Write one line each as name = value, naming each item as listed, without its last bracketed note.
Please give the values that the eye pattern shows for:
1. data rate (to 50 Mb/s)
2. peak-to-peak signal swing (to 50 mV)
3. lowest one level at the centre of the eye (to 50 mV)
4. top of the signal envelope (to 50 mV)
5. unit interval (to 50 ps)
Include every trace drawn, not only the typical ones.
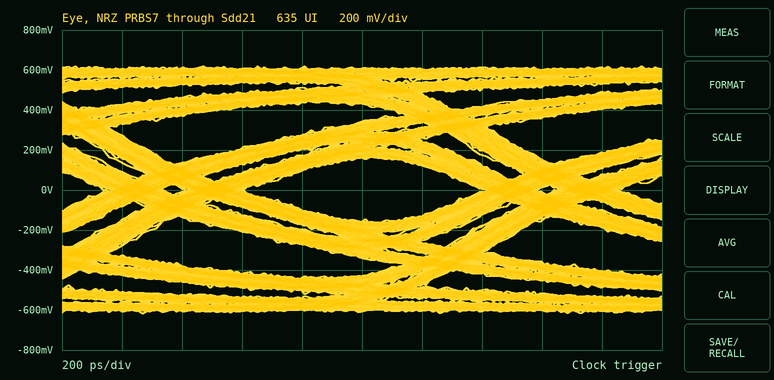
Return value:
data rate = 800 Mb/s
peak-to-peak signal swing = 1.25 V
lowest one level at the centre of the eye = 150 mV
top of the signal envelope = 600 mV
unit interval = 1.25 ns
